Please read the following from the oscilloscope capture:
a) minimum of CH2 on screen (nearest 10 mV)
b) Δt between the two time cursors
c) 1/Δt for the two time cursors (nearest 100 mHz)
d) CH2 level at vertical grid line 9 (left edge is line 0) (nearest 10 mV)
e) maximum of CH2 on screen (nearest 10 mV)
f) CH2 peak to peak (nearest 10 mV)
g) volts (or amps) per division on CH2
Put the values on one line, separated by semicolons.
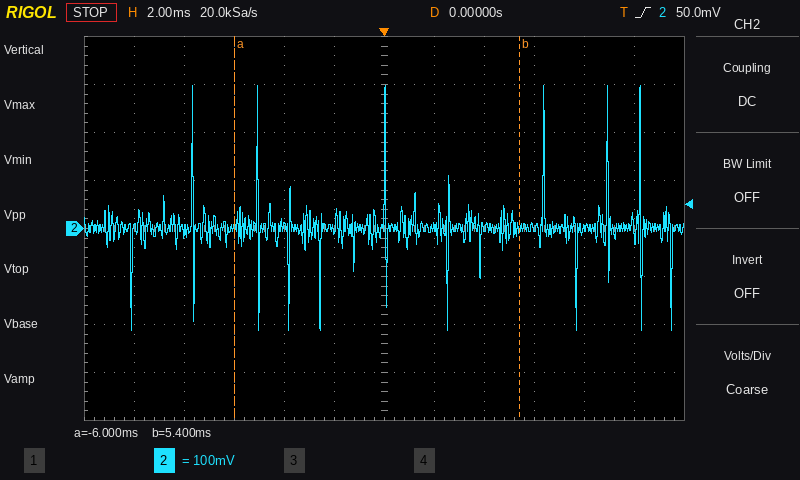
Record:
-210 mV; 11.4 ms; 87.7 Hz; 0 mV; 300 mV; 510 mV; 100 mV
